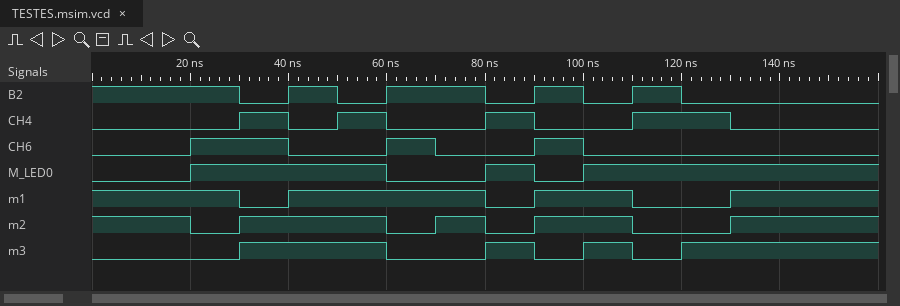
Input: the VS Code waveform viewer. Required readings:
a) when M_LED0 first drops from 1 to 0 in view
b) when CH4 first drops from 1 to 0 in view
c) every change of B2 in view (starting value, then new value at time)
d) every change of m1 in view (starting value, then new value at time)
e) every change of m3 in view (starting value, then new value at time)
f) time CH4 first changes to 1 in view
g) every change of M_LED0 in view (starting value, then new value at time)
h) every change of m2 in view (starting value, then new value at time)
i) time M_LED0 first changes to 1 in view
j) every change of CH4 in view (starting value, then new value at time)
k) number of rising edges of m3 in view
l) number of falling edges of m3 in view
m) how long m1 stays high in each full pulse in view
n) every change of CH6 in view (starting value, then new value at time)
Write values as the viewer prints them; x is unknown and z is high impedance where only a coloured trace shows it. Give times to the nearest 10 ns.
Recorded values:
60 ns
40 ns
1, 0 at 30 ns, 1 at 40 ns, 0 at 50 ns, 1 at 60 ns, 0 at 80 ns, 1 at 90 ns, 0 at 100 ns, 1 at 110 ns, 0 at 120 ns
1, 0 at 30 ns, 1 at 40 ns, 0 at 80 ns, 1 at 90 ns, 0 at 110 ns, 1 at 130 ns
0, 1 at 30 ns, 0 at 60 ns, 1 at 80 ns, 0 at 90 ns, 1 at 100 ns, 0 at 110 ns, 1 at 120 ns
30 ns
0, 1 at 20 ns, 0 at 60 ns, 1 at 80 ns, 0 at 90 ns, 1 at 100 ns
1, 0 at 20 ns, 1 at 30 ns, 0 at 60 ns, 1 at 70 ns, 0 at 80 ns, 1 at 90 ns, 0 at 110 ns, 1 at 130 ns
20 ns
0, 1 at 30 ns, 0 at 40 ns, 1 at 50 ns, 0 at 60 ns, 1 at 80 ns, 0 at 90 ns, 1 at 110 ns, 0 at 130 ns
4
3
40 ns, 20 ns
0, 1 at 20 ns, 0 at 40 ns, 1 at 60 ns, 0 at 70 ns, 1 at 90 ns, 0 at 100 ns
